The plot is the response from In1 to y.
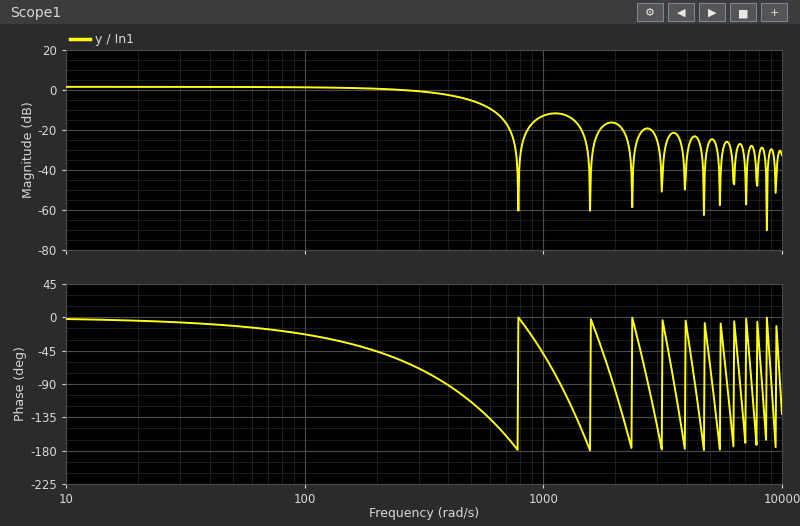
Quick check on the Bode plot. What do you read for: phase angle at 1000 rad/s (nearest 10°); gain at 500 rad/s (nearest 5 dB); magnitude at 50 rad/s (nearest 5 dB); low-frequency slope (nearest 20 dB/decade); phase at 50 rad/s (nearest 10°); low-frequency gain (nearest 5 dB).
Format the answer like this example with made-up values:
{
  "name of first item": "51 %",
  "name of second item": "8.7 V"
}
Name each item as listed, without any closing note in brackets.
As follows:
{
  "phase angle at 1000 rad/s": "-50°",
  "gain at 500 rad/s": "-5 dB",
  "magnitude at 50 rad/s": "0 dB",
  "low-frequency slope": "0 dB/decade",
  "phase at 50 rad/s": "-10°",
  "low-frequency gain": "0 dB"
}
